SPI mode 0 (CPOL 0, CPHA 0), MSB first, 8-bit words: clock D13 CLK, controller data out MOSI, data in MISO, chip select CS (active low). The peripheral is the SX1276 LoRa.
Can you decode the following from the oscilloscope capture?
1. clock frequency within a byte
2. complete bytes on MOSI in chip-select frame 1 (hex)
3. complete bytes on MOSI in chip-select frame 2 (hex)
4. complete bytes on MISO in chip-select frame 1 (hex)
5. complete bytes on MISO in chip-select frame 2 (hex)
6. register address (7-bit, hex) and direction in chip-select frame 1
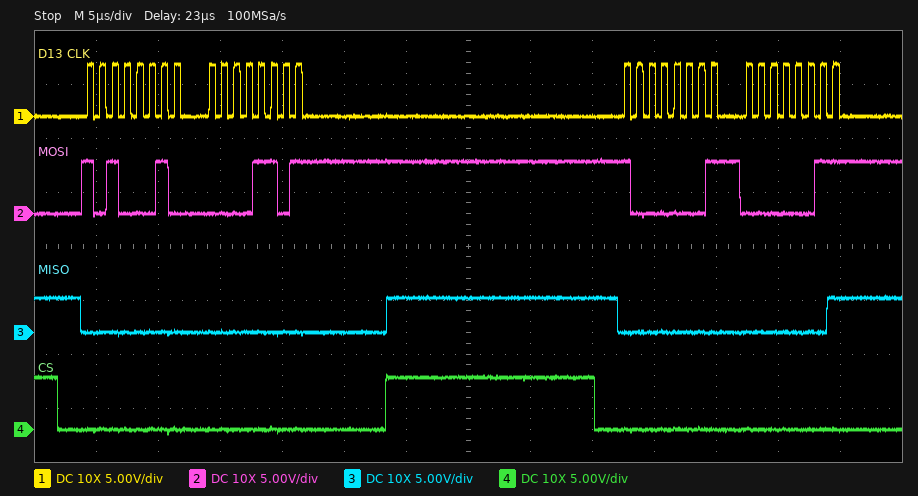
1 MHz
A2 0D
81 03
00 00
00 01
0x22 write
